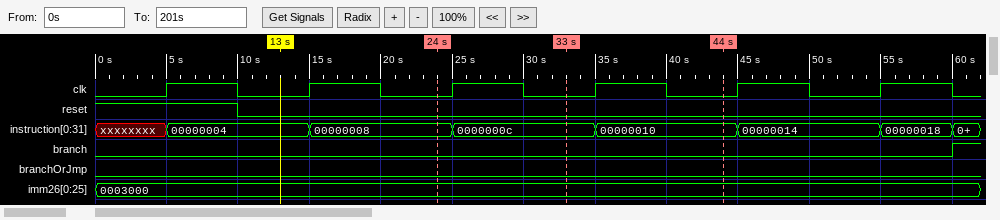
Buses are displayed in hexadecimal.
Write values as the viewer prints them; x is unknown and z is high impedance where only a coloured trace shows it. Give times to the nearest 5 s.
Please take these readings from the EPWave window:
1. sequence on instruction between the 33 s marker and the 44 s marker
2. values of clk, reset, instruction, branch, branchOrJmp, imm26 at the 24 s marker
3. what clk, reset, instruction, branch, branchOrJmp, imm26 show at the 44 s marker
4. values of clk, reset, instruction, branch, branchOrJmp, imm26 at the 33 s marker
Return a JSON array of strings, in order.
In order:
["0000000c, 00000010", "clk=0, reset=0, instruction=00000008, branch=0, branchOrJmp=0, imm26=0003000", "clk=0, reset=0, instruction=00000010, branch=0, branchOrJmp=0, imm26=0003000", "clk=0, reset=0, instruction=0000000c, branch=0, branchOrJmp=0, imm26=0003000"]
